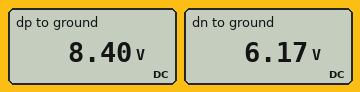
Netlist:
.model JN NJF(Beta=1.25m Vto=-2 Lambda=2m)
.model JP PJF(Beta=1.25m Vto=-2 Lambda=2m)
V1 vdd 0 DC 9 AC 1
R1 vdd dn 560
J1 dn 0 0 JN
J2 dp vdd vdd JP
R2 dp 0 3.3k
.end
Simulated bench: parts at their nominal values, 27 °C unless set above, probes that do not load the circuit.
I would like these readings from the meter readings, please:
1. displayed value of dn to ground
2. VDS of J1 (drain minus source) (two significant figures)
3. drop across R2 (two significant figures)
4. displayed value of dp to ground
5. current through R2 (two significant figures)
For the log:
6.17 V
6.2 V
8.4 V
8.40 V
2.5 mA
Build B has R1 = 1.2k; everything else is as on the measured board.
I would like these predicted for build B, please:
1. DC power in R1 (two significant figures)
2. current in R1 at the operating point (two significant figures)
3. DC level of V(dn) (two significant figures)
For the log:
30 mW
5.0 mA
3.0 V
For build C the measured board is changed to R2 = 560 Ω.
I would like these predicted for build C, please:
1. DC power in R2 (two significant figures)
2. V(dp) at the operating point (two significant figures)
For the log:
14 mW
2.8 V
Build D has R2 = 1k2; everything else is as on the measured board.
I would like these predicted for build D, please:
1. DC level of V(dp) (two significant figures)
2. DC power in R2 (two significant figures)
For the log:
6.0 V
30 mW
